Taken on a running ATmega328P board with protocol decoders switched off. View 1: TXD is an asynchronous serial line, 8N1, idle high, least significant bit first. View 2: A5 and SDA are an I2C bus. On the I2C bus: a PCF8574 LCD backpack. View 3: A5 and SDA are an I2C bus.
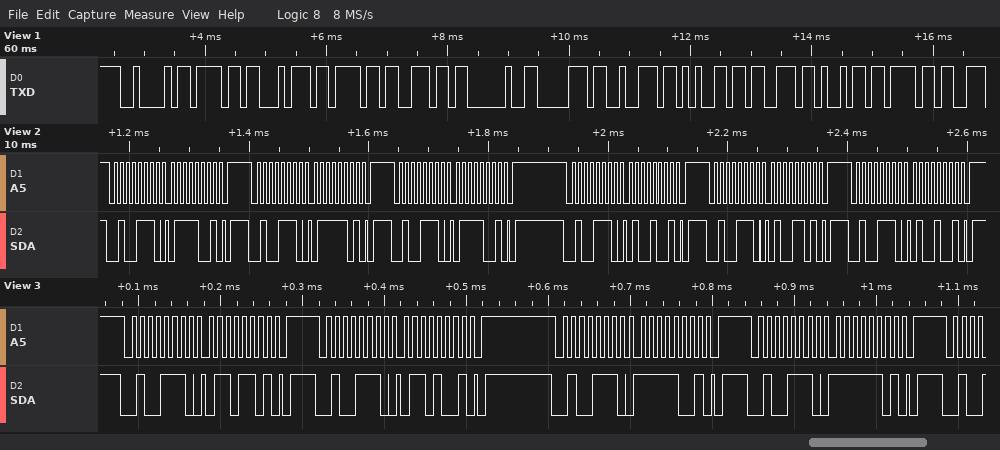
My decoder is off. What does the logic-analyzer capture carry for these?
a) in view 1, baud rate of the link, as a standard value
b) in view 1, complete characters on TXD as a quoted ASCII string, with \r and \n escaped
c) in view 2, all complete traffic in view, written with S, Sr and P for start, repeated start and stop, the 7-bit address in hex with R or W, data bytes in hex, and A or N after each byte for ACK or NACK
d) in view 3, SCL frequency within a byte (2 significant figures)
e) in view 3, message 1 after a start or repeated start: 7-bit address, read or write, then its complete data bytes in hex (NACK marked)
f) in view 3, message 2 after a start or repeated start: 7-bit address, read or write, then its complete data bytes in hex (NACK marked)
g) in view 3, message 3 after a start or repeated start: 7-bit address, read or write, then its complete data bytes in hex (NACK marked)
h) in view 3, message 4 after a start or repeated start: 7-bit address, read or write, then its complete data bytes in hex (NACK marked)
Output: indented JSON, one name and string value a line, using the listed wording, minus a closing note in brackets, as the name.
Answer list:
{
  "in view 1, baud rate of the link, as a standard value": "9600 baud",
  "in view 1, complete characters on TXD as a quoted ASCII string, with \\r and \\n escaped": "\"Boton presio\"",
  "in view 2, all complete traffic in view, written with S, Sr and P for start, repeated start and stop, the 7-bit address in hex with R or W, data bytes in hex, and A or N after each byte for ACK or NACK": "S 27W A 79 A P S 27W A 7D A P S 27W A 79 A P S 27W A 49 A P S 27W A 4D A P S 27W A 49 A P",
  "in view 3, SCL frequency within a byte": "100 kHz",
  "in view 3, message 1 after a start or repeated start: 7-bit address, read or write, then its complete data bytes in hex": "0x27 write: 6D",
  "in view 3, message 2 after a start or repeated start: 7-bit address, read or write, then its complete data bytes in hex": "0x27 write: 69",
  "in view 3, message 3 after a start or repeated start: 7-bit address, read or write, then its complete data bytes in hex": "0x27 write: F9",
  "in view 3, message 4 after a start or repeated start: 7-bit address, read or write, then its complete data bytes in hex": "0x27 write: FD"
}
